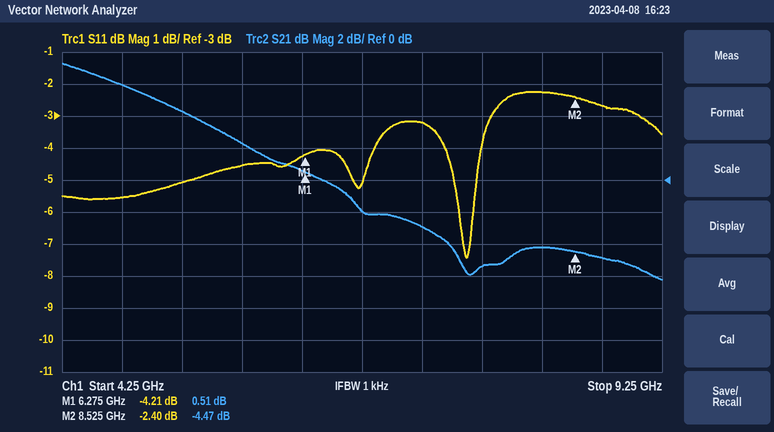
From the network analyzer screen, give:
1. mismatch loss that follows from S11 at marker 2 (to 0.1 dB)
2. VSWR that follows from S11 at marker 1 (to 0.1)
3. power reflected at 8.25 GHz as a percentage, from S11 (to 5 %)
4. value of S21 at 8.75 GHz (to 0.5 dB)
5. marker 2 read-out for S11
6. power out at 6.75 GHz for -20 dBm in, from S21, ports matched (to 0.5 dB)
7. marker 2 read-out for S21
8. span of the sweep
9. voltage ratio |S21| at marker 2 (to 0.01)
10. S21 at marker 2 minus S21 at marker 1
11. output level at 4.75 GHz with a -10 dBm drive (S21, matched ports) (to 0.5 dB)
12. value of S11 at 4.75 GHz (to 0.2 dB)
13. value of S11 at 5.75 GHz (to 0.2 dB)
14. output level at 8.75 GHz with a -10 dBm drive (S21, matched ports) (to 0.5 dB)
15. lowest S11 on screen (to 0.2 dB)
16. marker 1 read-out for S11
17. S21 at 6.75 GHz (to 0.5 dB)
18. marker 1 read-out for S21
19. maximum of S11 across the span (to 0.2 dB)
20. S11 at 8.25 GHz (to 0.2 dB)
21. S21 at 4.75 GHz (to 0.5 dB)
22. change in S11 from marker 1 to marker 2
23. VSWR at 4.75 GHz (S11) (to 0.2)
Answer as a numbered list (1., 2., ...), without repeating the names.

1. 3.7 dB
2. 4.2
3. 60 %
4. -5.0 dB
5. -2.40 dB
6. -22.0 dBm
7. -4.47 dB
8. 5 GHz
9. 0.60
10. -4.98 dB
11. -4.0 dBm
12. -5.6 dB
13. -4.6 dB
14. -15.0 dBm
15. -7.4 dB
16. -4.21 dB
17. -2.0 dB
18. 0.51 dB
19. -2.2 dB
20. -2.2 dB
21. 6.0 dB
22. 1.81 dB
23. 3.2
